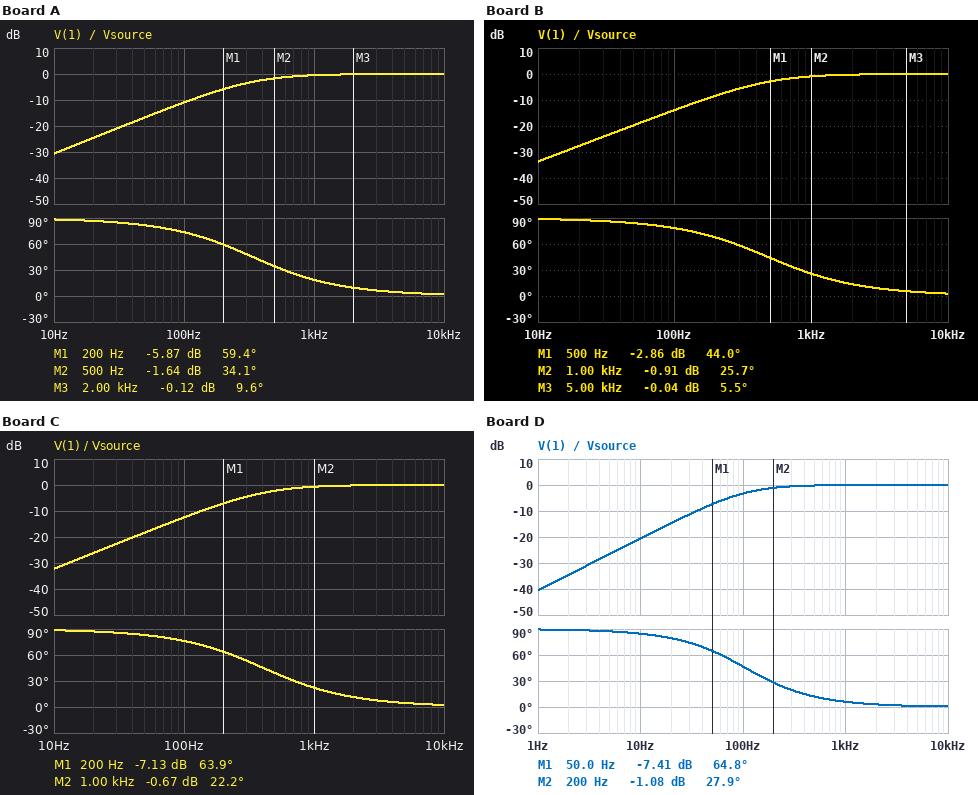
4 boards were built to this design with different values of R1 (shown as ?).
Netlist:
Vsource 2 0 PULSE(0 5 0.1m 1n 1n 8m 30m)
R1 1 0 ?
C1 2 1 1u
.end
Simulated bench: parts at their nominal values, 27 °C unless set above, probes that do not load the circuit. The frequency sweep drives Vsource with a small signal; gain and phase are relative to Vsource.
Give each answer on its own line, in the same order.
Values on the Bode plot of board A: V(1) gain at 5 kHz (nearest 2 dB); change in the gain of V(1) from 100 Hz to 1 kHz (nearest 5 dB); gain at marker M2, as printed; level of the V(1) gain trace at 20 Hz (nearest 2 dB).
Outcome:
0 dB
10 dB
-1.64 dB
-24 dB
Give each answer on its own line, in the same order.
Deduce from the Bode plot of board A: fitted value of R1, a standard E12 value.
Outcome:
470 Ω
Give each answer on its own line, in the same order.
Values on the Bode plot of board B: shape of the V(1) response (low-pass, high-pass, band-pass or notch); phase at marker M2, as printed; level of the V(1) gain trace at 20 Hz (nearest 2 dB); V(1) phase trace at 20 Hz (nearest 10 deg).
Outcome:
high-pass
25.7 deg
-28 dB
90 deg
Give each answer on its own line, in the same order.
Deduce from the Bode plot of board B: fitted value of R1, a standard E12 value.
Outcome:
330 Ω
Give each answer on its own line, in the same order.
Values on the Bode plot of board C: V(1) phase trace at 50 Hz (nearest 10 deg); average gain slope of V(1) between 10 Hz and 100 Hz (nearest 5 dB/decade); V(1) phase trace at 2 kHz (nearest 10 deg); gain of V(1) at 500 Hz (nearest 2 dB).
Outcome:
80 deg
20 dB/decade
10 deg
-2 dB
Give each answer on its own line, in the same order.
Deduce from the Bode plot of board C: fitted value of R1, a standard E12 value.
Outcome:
390 Ω
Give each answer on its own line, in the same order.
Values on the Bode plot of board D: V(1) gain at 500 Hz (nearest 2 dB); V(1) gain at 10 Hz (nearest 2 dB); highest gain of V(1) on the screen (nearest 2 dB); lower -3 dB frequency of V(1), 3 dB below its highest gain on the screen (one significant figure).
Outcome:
0 dB
-20 dB
0 dB
100 Hz
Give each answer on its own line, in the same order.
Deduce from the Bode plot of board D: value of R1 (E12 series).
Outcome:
1.5 kΩ
